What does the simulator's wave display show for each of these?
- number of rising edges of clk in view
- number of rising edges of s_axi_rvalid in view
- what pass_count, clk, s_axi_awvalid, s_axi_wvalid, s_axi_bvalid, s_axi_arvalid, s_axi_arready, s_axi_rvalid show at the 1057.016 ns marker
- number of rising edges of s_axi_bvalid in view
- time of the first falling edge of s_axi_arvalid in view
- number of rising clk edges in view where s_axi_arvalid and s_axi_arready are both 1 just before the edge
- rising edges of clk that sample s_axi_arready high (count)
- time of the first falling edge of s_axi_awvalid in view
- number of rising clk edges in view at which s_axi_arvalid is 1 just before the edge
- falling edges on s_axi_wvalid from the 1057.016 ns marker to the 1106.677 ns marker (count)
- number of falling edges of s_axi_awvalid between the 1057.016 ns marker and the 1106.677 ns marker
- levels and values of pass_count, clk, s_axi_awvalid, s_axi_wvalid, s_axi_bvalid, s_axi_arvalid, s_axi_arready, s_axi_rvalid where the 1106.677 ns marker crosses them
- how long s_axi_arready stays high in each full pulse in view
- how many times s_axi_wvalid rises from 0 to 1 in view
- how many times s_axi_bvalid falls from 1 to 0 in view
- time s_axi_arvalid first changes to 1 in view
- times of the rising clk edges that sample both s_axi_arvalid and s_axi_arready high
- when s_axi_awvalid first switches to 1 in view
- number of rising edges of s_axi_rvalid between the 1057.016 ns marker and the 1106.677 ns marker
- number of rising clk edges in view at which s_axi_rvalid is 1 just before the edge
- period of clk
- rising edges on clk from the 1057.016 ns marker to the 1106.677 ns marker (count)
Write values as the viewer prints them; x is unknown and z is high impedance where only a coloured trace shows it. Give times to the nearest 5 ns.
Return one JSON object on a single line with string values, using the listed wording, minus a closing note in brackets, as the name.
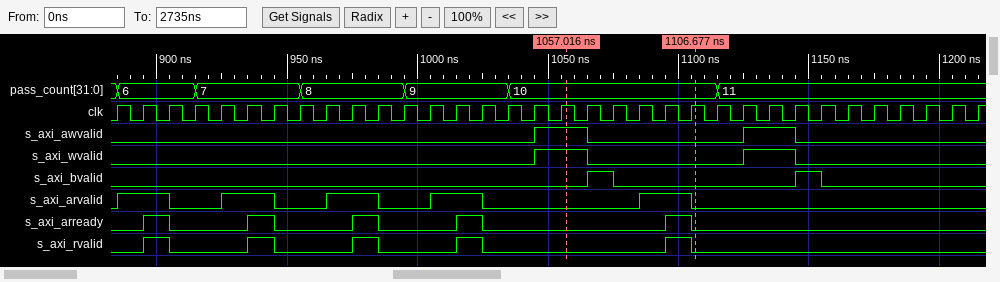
{"number of rising edges of clk in view": "34", "number of rising edges of s_axi_rvalid in view": "5", "what pass_count, clk, s_axi_awvalid, s_axi_wvalid, s_axi_bvalid, s_axi_arvalid, s_axi_arready, s_axi_rvalid show at the 1057.016 ns marker": "pass_count=10, clk=1, s_axi_awvalid=1, s_axi_wvalid=1, s_axi_bvalid=0, s_axi_arvalid=0, s_axi_arready=0, s_axi_rvalid=0", "number of rising edges of s_axi_bvalid in view": "2", "time of the first falling edge of s_axi_arvalid in view": "905 ns", "number of rising clk edges in view where s_axi_arvalid and s_axi_arready are both 1 just before the edge": "5", "rising edges of clk that sample s_axi_arready high": "5", "time of the first falling edge of s_axi_awvalid in view": "1065 ns", "number of rising clk edges in view at which s_axi_arvalid is 1 just before the edge": "10", "falling edges on s_axi_wvalid from the 1057.016 ns marker to the 1106.677 ns marker": "1", "number of falling edges of s_axi_awvalid between the 1057.016 ns marker and the 1106.677 ns marker": "1", "levels and values of pass_count, clk, s_axi_awvalid, s_axi_wvalid, s_axi_bvalid, s_axi_arvalid, s_axi_arready, s_axi_rvalid where the 1106.677 ns marker crosses them": "pass_count=10, clk=1, s_axi_awvalid=0, s_axi_wvalid=0, s_axi_bvalid=0, s_axi_arvalid=0, s_axi_arready=0, s_axi_rvalid=0", "how long s_axi_arready stays high in each full pulse in view": "10 ns, 10 ns, 10 ns, 10 ns, 10 ns", "how many times s_axi_wvalid rises from 0 to 1 in view": "2", "how many times s_axi_bvalid falls from 1 to 0 in view": "2", "time s_axi_arvalid first changes to 1 in view": "885 ns", "times of the rising clk edges that sample both s_axi_arvalid and s_axi_arready high": "905 ns, 945 ns, 985 ns, 1025 ns, 1105 ns", "when s_axi_awvalid first switches to 1 in view": "1045 ns", "number of rising edges of s_axi_rvalid between the 1057.016 ns marker and the 1106.677 ns marker": "1", "number of rising clk edges in view at which s_axi_rvalid is 1 just before the edge": "5", "period of clk": "10 ns", "rising edges on clk from the 1057.016 ns marker to the 1106.677 ns marker": "5"}
